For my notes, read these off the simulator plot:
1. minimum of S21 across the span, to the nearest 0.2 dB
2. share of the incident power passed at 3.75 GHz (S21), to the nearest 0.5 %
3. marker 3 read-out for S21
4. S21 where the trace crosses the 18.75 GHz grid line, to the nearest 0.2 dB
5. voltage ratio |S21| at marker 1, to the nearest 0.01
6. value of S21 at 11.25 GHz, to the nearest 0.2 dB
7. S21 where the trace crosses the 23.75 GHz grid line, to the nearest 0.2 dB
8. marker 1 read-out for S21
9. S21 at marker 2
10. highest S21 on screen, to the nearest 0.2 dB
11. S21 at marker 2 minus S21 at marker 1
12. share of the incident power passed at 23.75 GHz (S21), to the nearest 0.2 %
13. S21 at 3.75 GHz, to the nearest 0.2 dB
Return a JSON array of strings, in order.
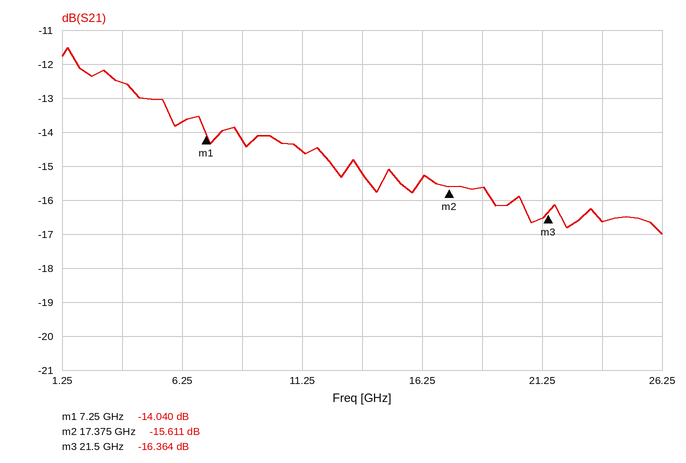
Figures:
["-17.0 dB", "5.5 %", "-16.364 dB", "-15.6 dB", "0.20", "-14.6 dB", "-16.6 dB", "-14.040 dB", "-15.611 dB", "-11.6 dB", "-1.571 dB", "2.2 %", "-12.6 dB"]
